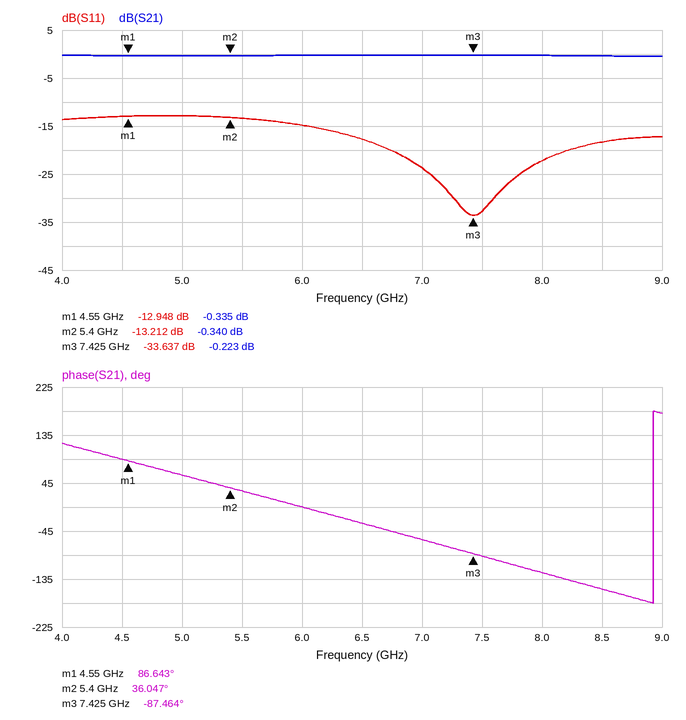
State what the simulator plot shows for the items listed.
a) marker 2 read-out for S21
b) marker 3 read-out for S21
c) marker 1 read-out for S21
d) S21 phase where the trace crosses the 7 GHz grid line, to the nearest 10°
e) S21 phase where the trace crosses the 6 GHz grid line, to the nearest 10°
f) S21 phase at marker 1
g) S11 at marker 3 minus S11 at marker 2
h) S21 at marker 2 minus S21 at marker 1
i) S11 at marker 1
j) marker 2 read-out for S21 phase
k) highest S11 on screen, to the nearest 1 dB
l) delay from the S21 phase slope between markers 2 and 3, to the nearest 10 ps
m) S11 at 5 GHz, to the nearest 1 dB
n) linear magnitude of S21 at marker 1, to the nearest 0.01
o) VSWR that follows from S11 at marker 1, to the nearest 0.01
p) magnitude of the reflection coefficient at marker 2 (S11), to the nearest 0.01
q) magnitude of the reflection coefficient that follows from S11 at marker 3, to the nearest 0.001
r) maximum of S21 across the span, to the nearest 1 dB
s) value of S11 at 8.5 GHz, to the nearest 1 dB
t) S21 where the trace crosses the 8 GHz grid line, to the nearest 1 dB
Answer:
-0.340 dB
-0.223 dB
-0.335 dB
-60°
0°
86.643°
-20.425 dB
-0.005 dB
-12.948 dB
36.047°
-13 dB
170 ps
-13 dB
0.96
1.58
0.22
0.021
0 dB
-18 dB
0 dB
